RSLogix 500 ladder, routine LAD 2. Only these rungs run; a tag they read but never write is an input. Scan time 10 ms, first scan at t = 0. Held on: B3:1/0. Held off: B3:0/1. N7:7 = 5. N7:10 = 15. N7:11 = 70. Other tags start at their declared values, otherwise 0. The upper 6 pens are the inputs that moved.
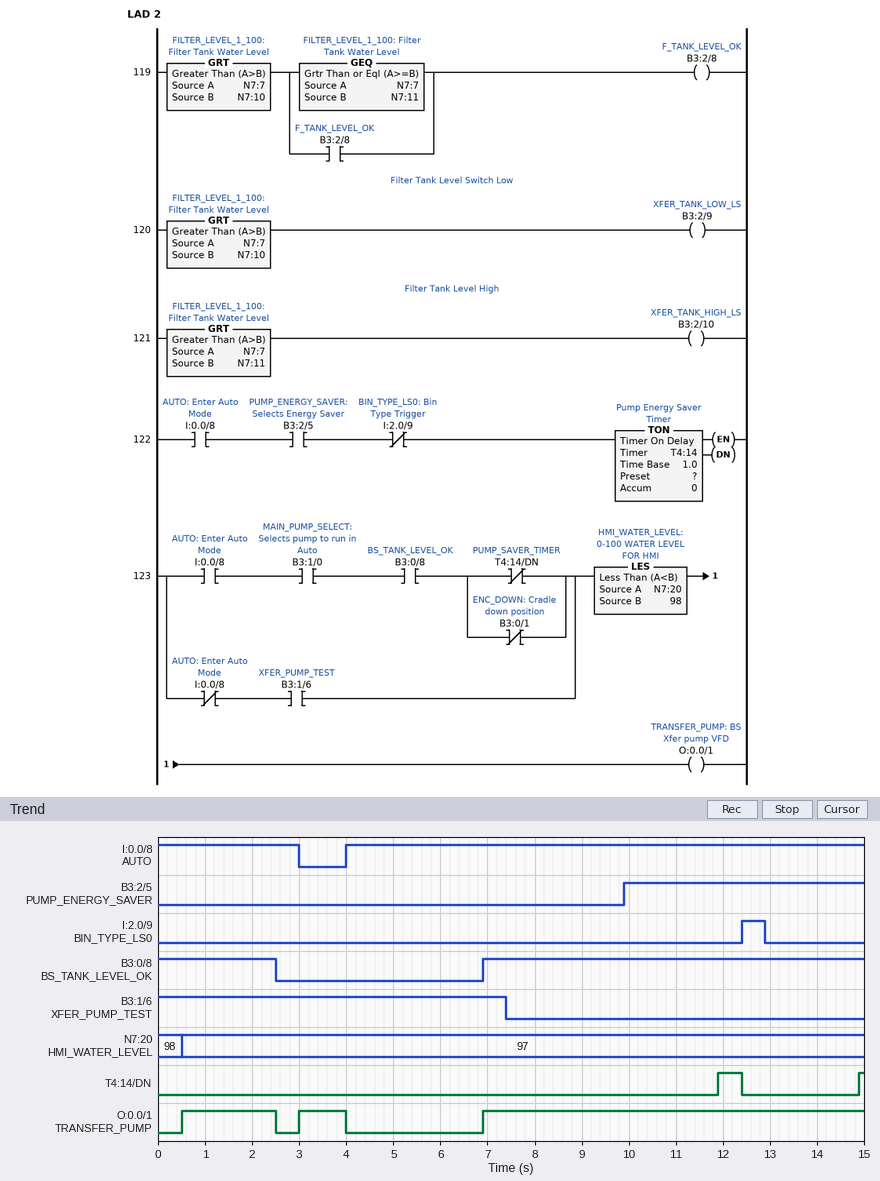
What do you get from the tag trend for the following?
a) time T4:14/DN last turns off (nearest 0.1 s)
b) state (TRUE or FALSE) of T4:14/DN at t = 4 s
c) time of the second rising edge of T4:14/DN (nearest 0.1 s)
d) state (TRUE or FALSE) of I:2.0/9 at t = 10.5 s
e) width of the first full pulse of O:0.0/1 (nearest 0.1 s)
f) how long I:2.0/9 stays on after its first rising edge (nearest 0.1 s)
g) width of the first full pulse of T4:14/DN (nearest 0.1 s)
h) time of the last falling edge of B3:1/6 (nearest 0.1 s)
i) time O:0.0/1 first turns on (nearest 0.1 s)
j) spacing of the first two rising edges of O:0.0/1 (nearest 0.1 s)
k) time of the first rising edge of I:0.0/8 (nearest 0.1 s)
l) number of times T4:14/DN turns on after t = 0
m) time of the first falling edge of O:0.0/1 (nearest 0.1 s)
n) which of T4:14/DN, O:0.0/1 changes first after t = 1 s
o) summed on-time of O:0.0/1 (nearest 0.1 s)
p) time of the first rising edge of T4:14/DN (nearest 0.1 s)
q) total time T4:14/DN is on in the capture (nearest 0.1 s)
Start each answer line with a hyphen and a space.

- 12.4 s
- FALSE
- 14.9 s
- FALSE
- 2.0 s
- 0.5 s
- 0.5 s
- 7.4 s
- 0.5 s
- 2.5 s
- 4.0 s
- 2
- 2.5 s
- O:0.0/1
- 11.1 s
- 11.9 s
- 0.6 s
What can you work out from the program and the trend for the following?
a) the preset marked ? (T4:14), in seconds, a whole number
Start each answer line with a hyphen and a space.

- 2 s
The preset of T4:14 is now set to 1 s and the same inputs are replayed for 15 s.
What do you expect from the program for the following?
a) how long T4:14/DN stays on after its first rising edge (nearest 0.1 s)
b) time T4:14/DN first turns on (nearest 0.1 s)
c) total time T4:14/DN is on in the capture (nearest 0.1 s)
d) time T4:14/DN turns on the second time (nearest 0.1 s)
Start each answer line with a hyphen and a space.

- 1.5 s
- 10.9 s
- 2.6 s
- 13.9 s
